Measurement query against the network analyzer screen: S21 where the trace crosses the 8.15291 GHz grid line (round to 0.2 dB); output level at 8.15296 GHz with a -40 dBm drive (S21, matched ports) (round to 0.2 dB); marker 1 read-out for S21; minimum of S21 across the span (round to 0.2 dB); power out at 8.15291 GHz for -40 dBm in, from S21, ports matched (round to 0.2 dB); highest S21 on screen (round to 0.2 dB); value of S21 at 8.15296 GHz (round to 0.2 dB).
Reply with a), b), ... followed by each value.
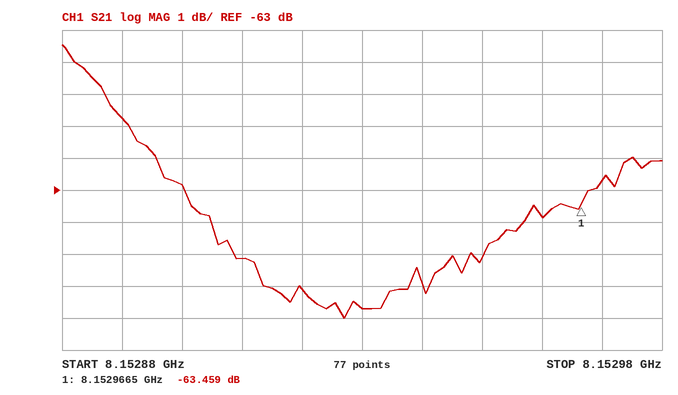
a) -65.2 dB
b) -103.8 dBm
c) -63.459 dB
d) -67.0 dB
e) -105.2 dBm
f) -58.4 dB
g) -63.8 dB
